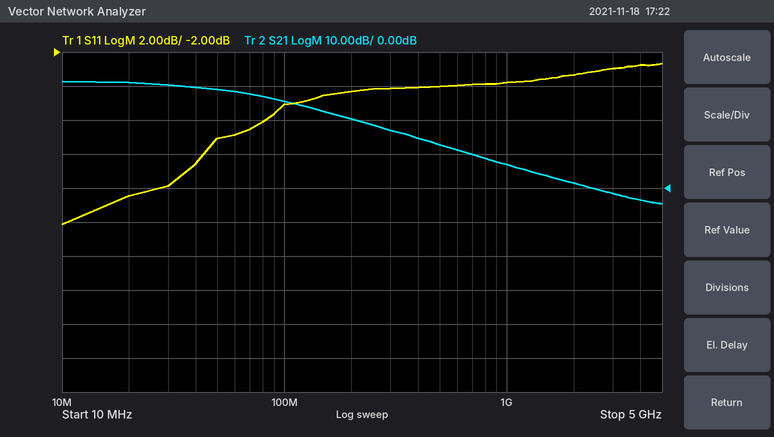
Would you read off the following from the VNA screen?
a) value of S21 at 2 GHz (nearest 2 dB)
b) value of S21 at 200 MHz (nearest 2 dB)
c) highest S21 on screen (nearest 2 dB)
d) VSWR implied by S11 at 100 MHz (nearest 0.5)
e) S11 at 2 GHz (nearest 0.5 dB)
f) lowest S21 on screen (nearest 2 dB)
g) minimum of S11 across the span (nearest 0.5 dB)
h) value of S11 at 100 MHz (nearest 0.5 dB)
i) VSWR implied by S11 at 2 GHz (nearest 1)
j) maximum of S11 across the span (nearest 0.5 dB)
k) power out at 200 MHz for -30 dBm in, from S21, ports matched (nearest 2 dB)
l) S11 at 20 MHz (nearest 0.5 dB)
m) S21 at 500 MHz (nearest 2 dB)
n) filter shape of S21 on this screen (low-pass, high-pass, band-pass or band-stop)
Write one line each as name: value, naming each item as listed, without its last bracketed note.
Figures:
value of S21 at 2 GHz: 2 dB
value of S21 at 200 MHz: 20 dB
highest S21 on screen: 32 dB
VSWR implied by S11 at 100 MHz: 3.5
S11 at 2 GHz: -3.5 dB
lowest S21 on screen: -4 dB
minimum of S11 across the span: -12.0 dB
value of S11 at 100 MHz: -5.0 dB
VSWR implied by S11 at 2 GHz: 5
maximum of S11 across the span: -2.5 dB
power out at 200 MHz for -30 dBm in, from S21, ports matched: -10 dBm
S11 at 20 MHz: -10.5 dB
S21 at 500 MHz: 12 dB
filter shape of S21 on this screen: low-pass
